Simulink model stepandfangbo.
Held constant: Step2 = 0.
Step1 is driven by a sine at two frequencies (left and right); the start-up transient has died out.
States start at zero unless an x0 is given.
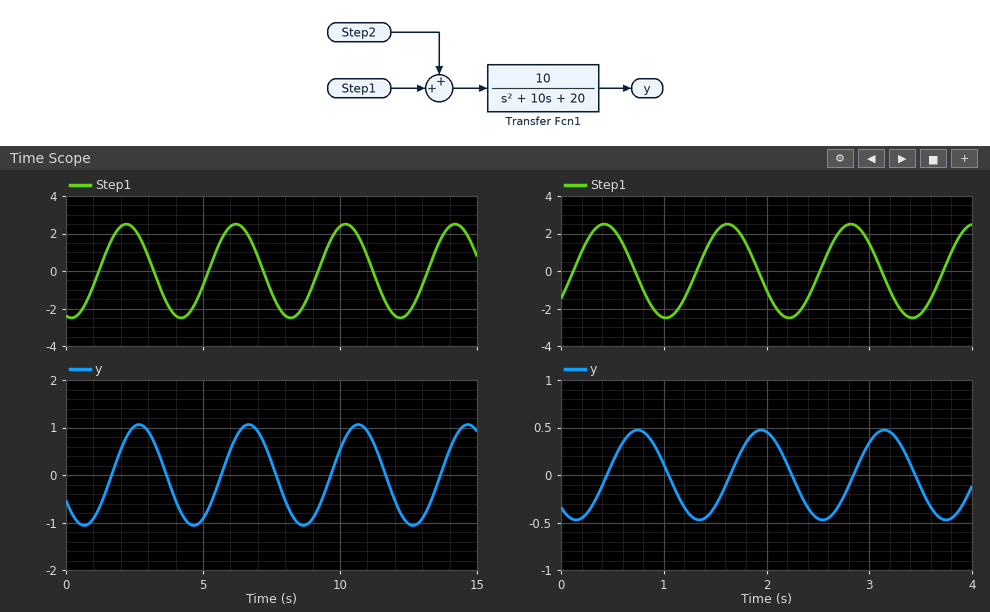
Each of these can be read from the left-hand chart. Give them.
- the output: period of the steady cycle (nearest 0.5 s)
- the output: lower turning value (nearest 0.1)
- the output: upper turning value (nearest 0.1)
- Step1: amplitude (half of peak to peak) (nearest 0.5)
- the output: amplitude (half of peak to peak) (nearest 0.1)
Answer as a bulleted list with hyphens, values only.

- 4.0 s
- -1.1
- 1.1
- 2.5
- 1.1
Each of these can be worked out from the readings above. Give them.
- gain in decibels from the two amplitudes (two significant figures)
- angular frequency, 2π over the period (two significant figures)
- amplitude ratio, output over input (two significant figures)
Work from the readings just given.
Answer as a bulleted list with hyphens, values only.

- -7.1 dB
- 1.6 rad/s
- 0.44
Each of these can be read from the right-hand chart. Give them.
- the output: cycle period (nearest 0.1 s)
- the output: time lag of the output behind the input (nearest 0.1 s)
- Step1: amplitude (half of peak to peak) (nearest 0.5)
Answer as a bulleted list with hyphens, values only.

- 1.2 s
- 0.3 s
- 2.5
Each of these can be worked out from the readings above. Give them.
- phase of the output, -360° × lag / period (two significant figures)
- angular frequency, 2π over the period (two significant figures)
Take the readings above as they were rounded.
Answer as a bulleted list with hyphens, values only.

- -90°
- 5.2 rad/s
